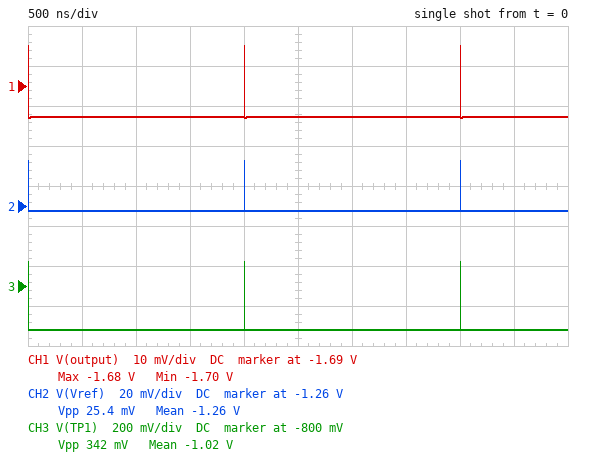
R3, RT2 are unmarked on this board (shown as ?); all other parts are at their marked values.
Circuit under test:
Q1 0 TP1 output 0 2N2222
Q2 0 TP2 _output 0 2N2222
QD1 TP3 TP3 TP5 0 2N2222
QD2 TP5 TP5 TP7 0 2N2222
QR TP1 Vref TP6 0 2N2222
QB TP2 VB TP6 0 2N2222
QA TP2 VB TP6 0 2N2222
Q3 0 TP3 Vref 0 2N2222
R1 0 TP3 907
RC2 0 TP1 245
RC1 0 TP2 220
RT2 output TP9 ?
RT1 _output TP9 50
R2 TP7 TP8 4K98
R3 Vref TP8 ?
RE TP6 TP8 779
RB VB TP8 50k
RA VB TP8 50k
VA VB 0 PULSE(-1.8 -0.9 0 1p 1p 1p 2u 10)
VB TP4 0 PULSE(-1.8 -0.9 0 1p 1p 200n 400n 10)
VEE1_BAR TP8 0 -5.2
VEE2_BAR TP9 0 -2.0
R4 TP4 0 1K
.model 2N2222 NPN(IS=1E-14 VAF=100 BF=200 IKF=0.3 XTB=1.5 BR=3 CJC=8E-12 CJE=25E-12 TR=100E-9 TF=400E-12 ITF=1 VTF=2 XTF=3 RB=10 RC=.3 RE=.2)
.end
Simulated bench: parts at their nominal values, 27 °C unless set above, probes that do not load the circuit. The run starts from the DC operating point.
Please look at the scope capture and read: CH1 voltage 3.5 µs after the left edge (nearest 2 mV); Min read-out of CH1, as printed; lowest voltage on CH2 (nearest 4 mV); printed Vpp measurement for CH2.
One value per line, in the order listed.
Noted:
-1.698 V
-1.70 V
-1.264 V
25.4 mV
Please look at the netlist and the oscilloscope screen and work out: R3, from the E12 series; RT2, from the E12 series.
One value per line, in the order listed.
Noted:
3.9 kΩ
120 Ω
